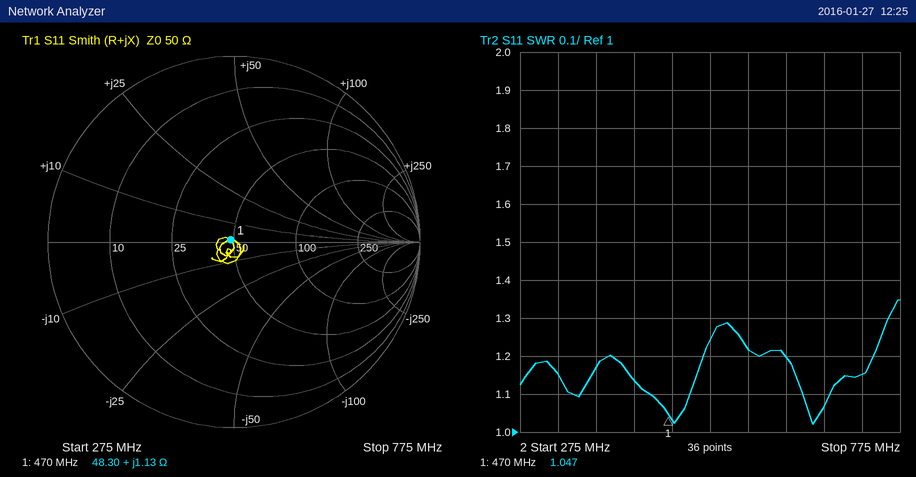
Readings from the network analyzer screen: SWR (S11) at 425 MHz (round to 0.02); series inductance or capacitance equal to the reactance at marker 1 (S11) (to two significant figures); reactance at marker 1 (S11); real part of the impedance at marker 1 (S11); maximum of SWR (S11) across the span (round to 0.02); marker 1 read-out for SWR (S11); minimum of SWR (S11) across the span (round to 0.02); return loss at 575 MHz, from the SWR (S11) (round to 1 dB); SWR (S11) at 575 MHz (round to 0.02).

1.14
380 pH
+1.13 Ω
48.30 Ω
1.34
1.047
1.02
20 dB
1.22
